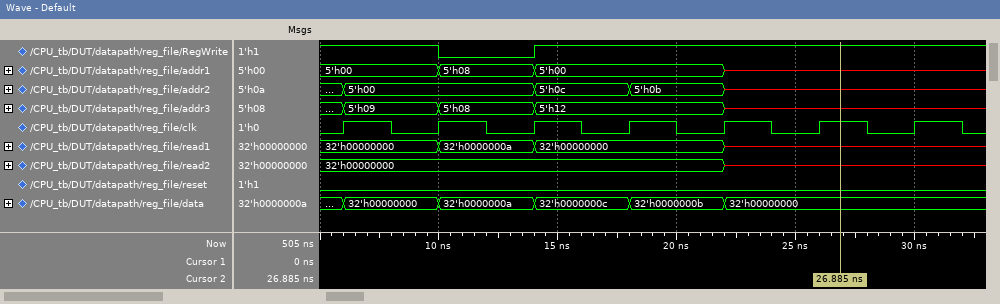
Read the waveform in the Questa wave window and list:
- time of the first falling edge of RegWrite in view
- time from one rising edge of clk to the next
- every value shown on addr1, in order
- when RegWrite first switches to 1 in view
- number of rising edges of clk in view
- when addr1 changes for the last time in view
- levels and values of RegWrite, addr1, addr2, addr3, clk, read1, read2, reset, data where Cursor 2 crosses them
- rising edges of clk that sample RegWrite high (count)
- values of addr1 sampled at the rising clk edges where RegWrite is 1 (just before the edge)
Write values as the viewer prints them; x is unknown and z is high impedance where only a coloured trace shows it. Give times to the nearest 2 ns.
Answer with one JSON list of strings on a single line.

["10 ns", "4 ns", "5'h00, 5'h08, 5'h00, x", "14 ns", "7", "22 ns", "RegWrite=1, addr1=x, addr2=x, addr3=x, clk=1, read1=x, read2=x, reset=0, data=32'h00000000", "6", "5'h00, 5'h00, 5'h00, 5'h00, x, x"]
